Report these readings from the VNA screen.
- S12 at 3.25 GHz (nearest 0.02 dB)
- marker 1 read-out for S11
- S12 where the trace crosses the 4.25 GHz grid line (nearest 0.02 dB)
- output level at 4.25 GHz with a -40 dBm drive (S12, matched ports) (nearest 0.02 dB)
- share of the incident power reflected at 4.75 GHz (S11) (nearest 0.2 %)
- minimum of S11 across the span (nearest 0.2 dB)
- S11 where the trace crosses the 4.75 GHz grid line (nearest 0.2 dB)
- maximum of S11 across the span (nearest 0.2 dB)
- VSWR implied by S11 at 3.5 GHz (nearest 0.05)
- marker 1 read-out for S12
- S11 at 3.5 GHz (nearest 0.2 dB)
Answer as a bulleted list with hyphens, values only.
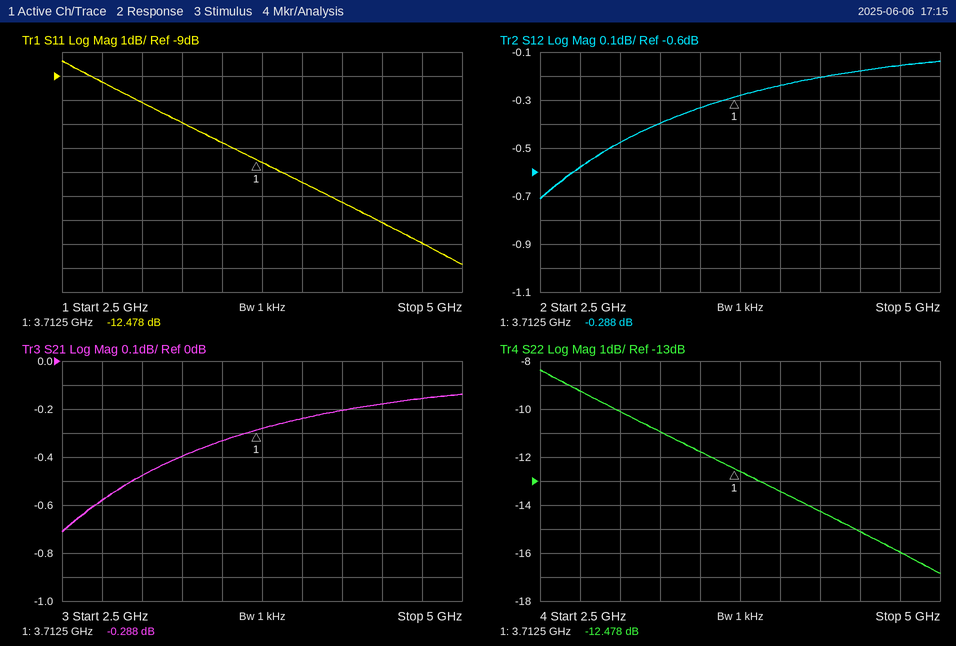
- -0.40 dB
- -12.478 dB
- -0.20 dB
- -40.20 dBm
- 2.6 %
- -16.8 dB
- -16.0 dB
- -8.4 dB
- 1.70
- -0.288 dB
- -11.8 dB
